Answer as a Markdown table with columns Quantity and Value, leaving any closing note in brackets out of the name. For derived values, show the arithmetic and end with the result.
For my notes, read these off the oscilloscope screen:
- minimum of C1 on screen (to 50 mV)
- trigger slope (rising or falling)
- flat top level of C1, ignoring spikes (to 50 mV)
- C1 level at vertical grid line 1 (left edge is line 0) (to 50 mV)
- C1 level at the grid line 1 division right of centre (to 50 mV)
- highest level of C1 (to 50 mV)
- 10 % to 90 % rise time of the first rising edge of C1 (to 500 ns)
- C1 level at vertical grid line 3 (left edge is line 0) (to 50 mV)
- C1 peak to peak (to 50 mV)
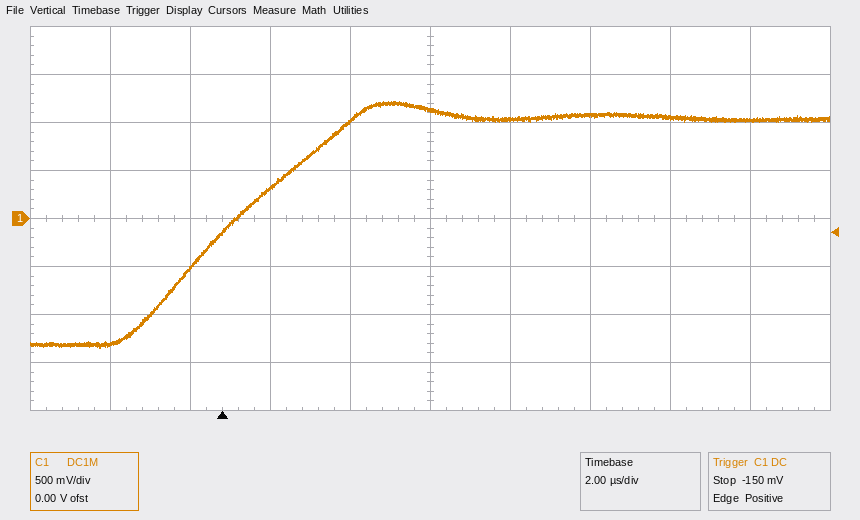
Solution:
| Quantity | Value |
|---|---|
| minimum of C1 on screen | -1.35 V |
| trigger slope | rising |
| flat top level of C1, ignoring spikes | 1.05 V |
| C1 level at vertical grid line 1 (left edge is line 0) | -1.30 V |
| C1 level at the grid line 1 division right of centre | 1.05 V |
| highest level of C1 | 1.20 V |
| 10 % to 90 % rise time of the first rising edge of C1 | 4.5 µs |
| C1 level at vertical grid line 3 (left edge is line 0) | 300 mV |
| C1 peak to peak | 1.20 V − (-1.35 V) = 2.55 V |
